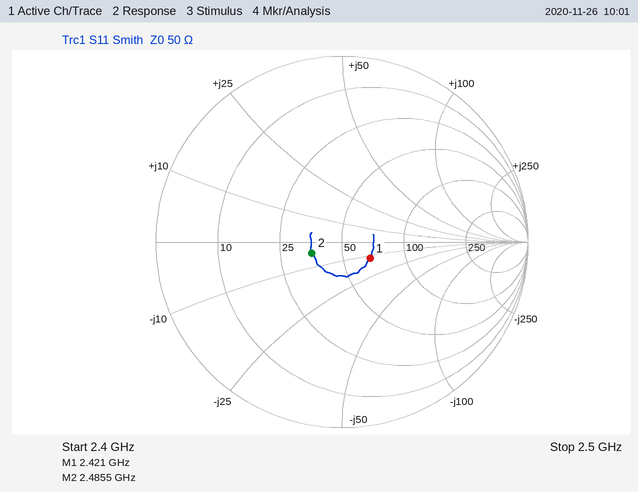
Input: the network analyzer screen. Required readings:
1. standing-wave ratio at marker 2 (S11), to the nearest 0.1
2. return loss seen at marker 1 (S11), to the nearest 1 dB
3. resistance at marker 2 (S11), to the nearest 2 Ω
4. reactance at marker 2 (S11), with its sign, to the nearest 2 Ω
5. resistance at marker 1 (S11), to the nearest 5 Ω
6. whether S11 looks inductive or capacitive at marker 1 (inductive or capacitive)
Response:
1.4
15 dB
36 Ω
-4 Ω
65 Ω
capacitive
